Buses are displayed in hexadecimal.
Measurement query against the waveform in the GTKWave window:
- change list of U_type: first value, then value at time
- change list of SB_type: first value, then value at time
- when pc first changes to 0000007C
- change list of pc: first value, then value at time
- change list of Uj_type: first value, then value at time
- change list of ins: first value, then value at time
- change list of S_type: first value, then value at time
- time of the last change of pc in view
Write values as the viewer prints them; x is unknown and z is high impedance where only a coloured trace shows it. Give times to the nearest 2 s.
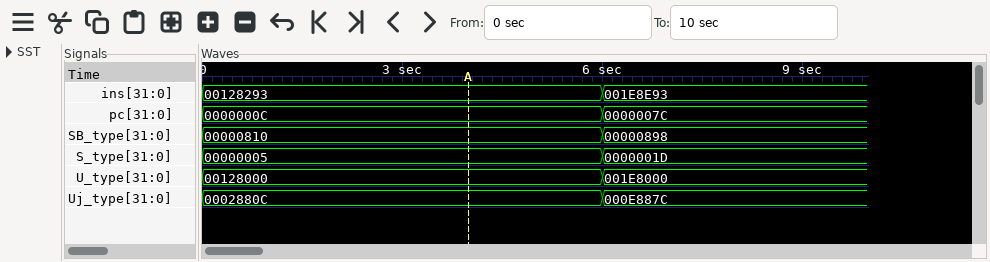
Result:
00128000, 001E8000 at 6 s
00000810, 00000898 at 6 s
6 s
0000000C, 0000007C at 6 s
0002880C, 000E887C at 6 s
00128293, 001E8E93 at 6 s
00000005, 0000001D at 6 s
6 s
